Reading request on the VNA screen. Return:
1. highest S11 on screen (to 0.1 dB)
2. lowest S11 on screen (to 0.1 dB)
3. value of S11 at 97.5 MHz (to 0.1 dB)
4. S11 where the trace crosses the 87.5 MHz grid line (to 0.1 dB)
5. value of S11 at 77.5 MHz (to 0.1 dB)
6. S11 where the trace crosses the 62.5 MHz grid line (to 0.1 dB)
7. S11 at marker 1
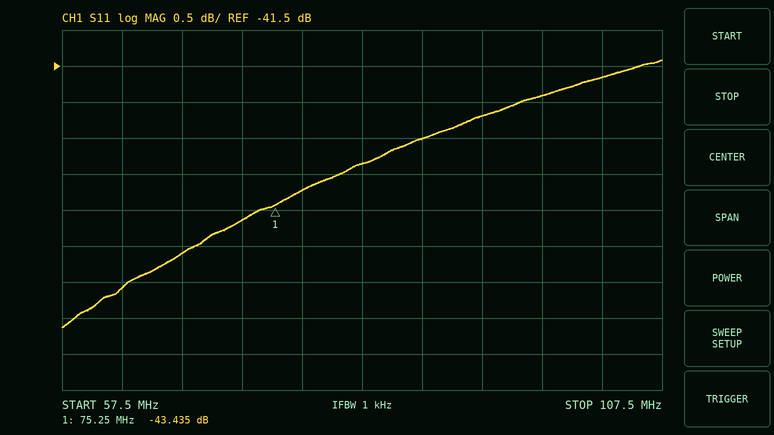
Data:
-41.4 dB
-45.1 dB
-41.9 dB
-42.5 dB
-43.2 dB
-44.6 dB
-43.435 dB
